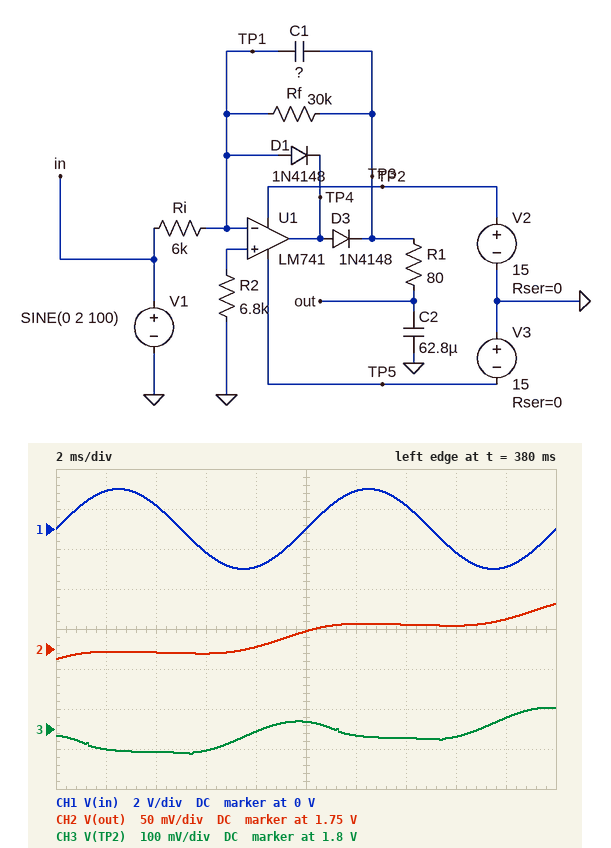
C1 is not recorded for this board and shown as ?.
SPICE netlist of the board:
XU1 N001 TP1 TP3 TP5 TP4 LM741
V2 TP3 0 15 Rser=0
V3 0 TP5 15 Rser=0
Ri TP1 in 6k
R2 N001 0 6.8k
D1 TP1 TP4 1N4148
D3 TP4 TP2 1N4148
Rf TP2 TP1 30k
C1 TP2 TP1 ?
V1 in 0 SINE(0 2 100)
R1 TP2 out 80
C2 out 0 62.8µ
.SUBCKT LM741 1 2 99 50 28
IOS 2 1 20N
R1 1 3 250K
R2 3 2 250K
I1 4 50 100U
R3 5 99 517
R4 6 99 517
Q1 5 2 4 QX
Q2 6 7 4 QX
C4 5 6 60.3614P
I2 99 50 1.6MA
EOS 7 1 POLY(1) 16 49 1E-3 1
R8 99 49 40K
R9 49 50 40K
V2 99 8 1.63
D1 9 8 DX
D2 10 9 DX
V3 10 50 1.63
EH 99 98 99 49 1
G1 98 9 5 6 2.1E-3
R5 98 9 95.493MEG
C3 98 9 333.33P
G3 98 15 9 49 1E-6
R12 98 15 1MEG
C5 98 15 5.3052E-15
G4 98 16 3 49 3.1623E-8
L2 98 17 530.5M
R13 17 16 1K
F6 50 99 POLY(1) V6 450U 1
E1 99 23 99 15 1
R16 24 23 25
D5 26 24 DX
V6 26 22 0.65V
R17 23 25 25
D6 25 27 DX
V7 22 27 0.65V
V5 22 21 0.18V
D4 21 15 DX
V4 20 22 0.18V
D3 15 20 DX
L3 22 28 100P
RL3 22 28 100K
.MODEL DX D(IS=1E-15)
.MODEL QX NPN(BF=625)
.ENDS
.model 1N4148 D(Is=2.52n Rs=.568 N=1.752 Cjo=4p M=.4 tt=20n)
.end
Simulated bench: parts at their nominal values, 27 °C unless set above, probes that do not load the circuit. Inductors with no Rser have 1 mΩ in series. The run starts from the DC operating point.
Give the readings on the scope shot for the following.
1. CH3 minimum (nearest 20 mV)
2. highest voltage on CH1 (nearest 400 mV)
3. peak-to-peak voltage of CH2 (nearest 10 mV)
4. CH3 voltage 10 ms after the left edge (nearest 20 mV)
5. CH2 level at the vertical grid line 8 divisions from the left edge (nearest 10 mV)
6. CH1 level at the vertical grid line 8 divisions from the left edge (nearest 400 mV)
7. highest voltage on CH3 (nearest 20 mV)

1.74 V
2.0 V
70 mV
1.82 V
1.78 V
-1.2 V
1.86 V
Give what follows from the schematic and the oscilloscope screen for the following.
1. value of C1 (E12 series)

10 µF
